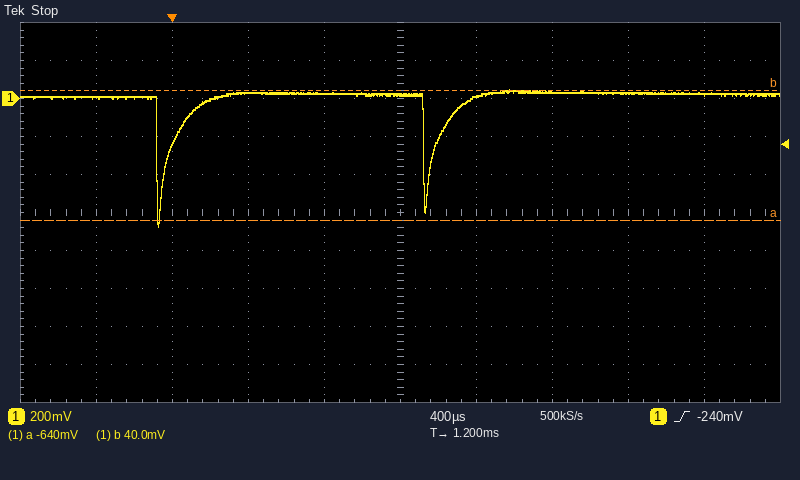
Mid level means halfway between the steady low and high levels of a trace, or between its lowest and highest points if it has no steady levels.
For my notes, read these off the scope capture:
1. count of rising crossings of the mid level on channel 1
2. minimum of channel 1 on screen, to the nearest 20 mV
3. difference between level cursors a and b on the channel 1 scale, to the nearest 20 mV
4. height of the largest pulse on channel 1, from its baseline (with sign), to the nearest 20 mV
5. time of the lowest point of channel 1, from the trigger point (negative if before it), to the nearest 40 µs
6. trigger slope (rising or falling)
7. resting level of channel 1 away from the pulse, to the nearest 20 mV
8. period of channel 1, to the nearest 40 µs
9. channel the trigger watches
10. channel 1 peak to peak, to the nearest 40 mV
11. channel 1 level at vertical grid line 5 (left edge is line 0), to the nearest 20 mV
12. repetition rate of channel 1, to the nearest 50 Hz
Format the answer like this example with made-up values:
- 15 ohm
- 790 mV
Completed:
- 2
- -680 mV
- 680 mV
- -700 mV
- -80 µs
- rising
- 20 mV
- 1.40 ms
- channel 1
- 720 mV
- 20 mV
- 700 Hz
